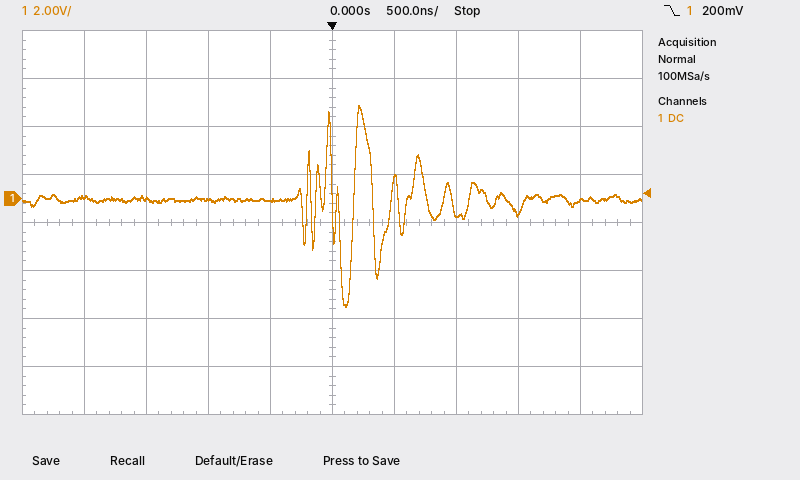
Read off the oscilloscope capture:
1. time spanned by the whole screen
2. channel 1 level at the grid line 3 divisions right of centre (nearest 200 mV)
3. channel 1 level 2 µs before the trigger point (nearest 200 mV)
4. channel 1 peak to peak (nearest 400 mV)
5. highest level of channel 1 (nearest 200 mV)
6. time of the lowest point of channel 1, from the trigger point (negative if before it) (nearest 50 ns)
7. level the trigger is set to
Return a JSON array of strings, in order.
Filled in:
["5 µs", "-600 mV", "0.0 V", "8.4 V", "3.8 V", "+100 ns", "200 mV"]
